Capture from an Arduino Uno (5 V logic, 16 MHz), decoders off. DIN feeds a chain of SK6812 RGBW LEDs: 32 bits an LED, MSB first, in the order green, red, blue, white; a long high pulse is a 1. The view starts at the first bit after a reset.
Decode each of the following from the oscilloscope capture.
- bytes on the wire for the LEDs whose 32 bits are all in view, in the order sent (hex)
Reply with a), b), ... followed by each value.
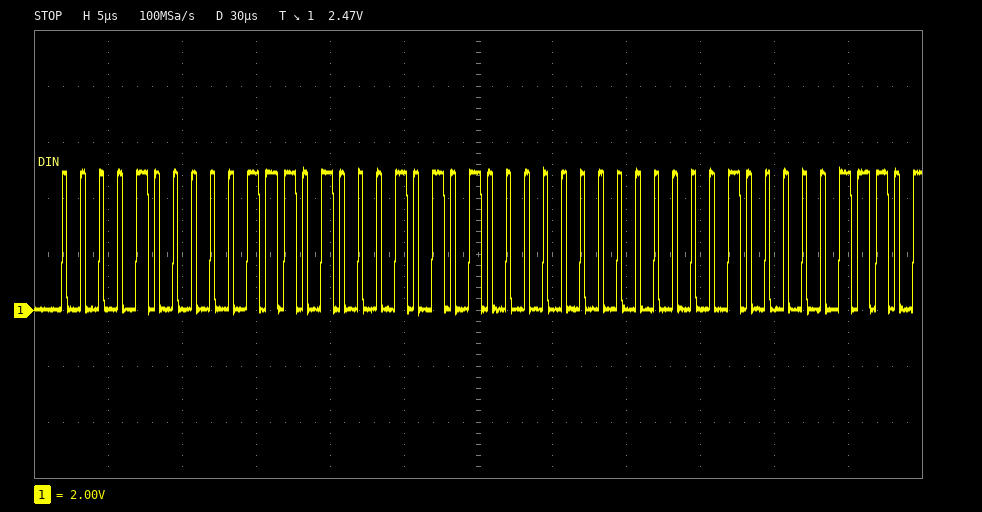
a) 08 3A 2A 00
